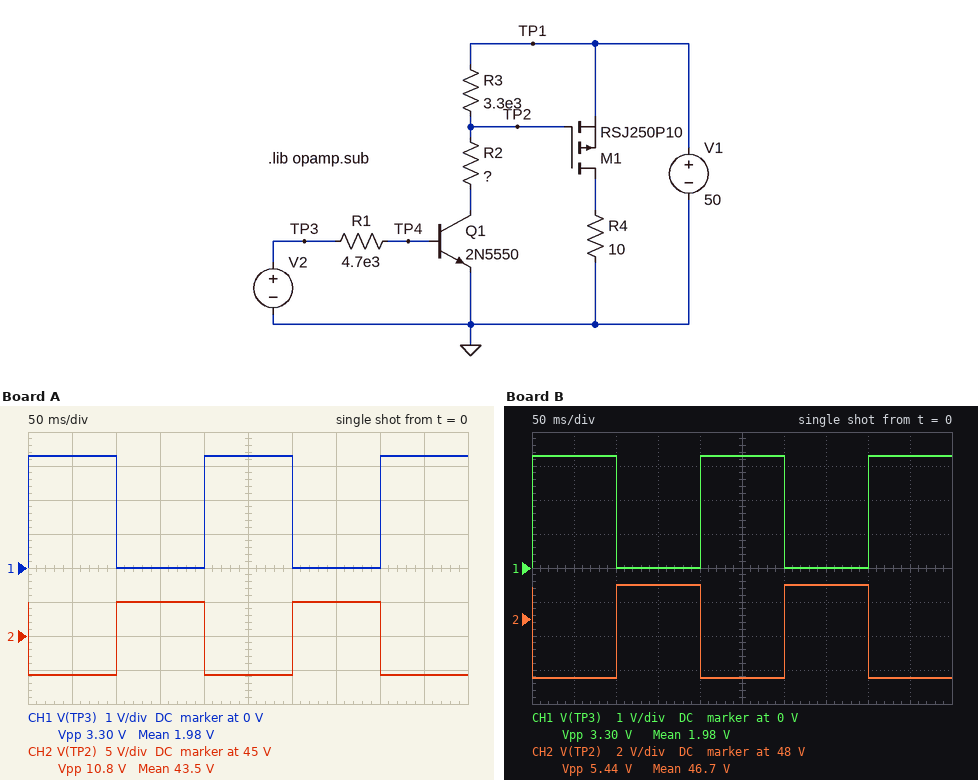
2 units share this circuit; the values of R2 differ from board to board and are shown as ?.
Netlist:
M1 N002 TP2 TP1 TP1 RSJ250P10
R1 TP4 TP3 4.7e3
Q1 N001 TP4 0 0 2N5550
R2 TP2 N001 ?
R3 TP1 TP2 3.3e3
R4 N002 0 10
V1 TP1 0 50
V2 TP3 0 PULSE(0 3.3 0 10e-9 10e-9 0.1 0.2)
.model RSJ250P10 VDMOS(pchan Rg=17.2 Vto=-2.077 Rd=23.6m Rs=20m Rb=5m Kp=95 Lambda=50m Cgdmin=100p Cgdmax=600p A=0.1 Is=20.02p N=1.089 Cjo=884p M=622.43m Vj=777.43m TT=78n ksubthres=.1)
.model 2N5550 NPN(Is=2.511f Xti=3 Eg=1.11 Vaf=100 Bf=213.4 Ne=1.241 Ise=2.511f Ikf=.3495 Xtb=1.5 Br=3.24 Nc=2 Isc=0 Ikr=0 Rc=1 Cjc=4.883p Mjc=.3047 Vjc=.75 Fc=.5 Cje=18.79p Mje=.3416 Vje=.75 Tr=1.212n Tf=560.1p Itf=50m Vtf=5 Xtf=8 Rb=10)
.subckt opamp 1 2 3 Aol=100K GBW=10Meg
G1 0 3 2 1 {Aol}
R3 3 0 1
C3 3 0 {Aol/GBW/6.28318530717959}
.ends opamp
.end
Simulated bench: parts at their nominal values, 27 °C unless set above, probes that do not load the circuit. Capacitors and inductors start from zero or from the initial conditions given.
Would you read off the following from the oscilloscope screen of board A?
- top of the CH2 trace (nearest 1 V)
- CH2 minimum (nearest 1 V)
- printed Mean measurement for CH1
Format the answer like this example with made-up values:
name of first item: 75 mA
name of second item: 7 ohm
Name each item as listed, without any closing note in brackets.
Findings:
top of the CH2 trace: 50 V
CH2 minimum: 39 V
printed Mean measurement for CH1: 1.98 V
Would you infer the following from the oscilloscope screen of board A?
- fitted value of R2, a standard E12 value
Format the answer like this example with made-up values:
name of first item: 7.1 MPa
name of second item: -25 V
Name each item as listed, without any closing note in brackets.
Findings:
fitted value of R2, a standard E12 value: 12 kΩ
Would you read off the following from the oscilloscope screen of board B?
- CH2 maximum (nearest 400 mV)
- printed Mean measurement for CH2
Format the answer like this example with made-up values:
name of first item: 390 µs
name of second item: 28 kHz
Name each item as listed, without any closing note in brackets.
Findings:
CH2 maximum: 50.0 V
printed Mean measurement for CH2: 46.7 V
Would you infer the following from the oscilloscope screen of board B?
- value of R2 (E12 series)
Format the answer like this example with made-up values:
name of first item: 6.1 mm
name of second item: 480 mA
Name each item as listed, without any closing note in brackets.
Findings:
value of R2: 27 kΩ
